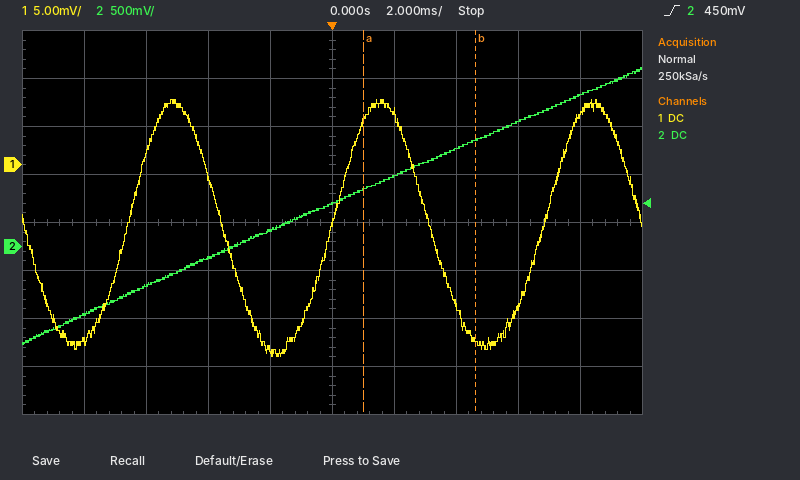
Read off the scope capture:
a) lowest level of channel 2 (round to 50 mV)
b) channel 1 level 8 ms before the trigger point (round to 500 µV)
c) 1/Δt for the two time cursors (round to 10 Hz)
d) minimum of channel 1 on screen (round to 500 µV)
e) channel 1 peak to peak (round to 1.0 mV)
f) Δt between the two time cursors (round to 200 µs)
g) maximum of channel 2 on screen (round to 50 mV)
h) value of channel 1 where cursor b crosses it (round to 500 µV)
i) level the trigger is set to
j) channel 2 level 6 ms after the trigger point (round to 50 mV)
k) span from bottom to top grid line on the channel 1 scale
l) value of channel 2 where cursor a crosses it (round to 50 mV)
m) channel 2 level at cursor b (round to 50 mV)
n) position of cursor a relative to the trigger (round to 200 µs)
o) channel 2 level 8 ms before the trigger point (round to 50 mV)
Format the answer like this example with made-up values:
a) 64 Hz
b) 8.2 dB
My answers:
a) -1.00 V
b) -18.5 mV
c) 280 Hz
d) -20.0 mV
e) 27.0 mV
f) 3.6 ms
g) 1.85 V
h) -18.5 mV
i) 450 mV
j) 1.30 V
k) 40 mV
l) 600 mV
m) 1.10 V
n) +1.0 ms
o) -700 mV
